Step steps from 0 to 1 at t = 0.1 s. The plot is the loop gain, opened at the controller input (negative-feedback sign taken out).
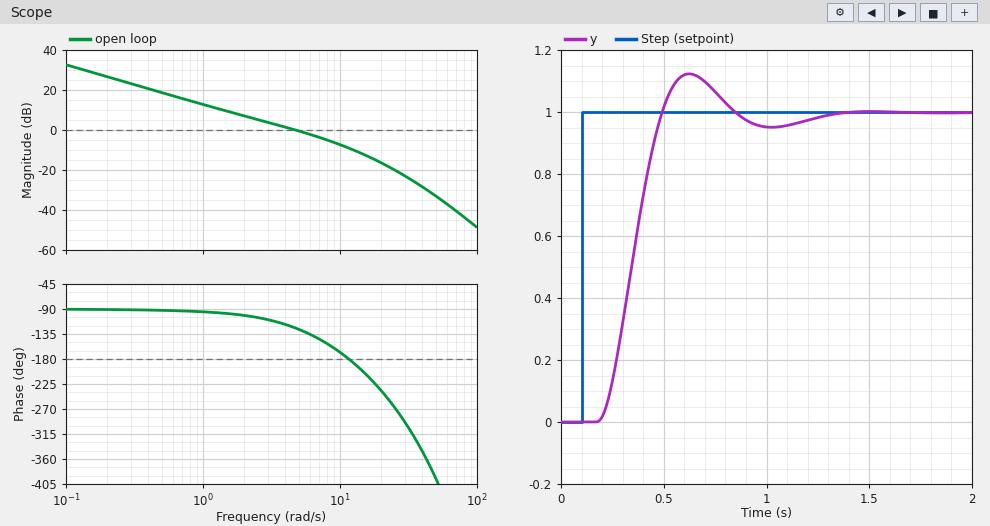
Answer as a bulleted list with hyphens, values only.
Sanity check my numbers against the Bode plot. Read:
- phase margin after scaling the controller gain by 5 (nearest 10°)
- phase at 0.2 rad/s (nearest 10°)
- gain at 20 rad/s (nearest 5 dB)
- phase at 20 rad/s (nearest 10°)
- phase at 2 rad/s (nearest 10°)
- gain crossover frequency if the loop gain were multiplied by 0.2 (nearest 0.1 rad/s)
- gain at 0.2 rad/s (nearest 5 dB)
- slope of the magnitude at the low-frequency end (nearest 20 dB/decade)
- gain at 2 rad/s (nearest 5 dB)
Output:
- -40°
- -90°
- -15 dB
- -240°
- -100°
- 0.9 rad/s
- 25 dB
- -20 dB/decade
- 5 dB
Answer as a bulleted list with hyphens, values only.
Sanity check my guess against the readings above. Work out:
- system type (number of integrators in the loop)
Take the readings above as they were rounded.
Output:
- 1
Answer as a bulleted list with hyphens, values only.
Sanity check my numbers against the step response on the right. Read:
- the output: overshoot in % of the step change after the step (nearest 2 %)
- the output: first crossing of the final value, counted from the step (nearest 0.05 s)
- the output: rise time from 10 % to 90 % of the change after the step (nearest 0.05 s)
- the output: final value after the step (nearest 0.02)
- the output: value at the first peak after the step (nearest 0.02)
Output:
- 12 %
- 0.40 s
- 0.20 s
- 1.00
- 1.12
